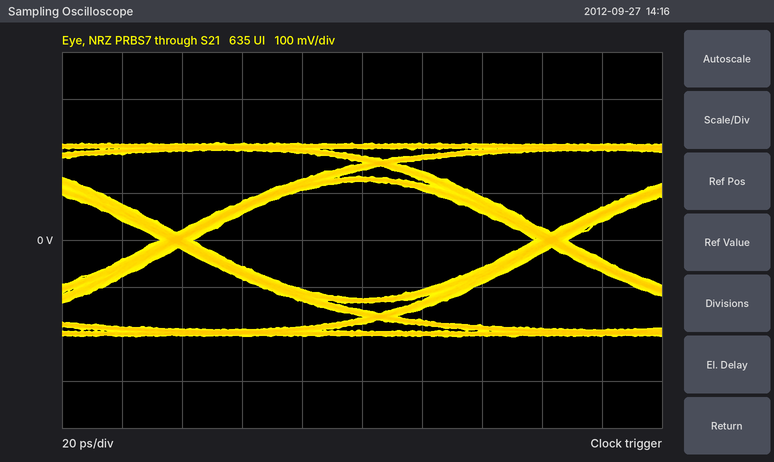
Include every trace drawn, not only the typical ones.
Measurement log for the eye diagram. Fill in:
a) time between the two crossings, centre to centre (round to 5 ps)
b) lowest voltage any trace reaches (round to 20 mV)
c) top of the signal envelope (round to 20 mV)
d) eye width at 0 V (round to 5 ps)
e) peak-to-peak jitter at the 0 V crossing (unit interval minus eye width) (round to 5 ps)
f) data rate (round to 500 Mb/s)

125 ps
-200 mV
200 mV
115 ps
10 ps
8.0 Gb/s
